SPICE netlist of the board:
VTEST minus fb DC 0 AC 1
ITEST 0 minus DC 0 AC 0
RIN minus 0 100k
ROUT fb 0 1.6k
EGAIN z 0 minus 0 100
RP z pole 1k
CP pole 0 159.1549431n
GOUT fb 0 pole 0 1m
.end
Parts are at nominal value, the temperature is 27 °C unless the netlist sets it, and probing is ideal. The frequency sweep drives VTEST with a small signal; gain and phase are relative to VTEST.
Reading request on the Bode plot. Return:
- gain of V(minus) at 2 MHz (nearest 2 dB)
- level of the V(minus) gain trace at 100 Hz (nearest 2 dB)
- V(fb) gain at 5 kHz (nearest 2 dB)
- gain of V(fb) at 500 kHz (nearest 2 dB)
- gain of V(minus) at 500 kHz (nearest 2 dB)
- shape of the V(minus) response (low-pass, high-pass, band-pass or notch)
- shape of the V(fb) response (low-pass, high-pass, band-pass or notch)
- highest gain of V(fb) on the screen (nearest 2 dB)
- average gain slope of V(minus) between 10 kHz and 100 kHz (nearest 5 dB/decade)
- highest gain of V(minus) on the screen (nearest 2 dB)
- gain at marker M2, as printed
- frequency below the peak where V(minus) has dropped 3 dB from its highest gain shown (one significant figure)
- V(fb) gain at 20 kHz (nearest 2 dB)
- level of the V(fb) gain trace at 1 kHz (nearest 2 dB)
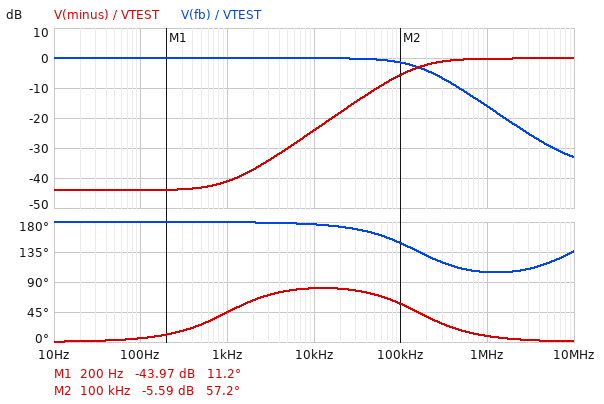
0 dB
-44 dB
0 dB
-10 dB
0 dB
high-pass
low-pass
0 dB
20 dB/decade
0 dB
-5.59 dB
200 kHz
0 dB
0 dB
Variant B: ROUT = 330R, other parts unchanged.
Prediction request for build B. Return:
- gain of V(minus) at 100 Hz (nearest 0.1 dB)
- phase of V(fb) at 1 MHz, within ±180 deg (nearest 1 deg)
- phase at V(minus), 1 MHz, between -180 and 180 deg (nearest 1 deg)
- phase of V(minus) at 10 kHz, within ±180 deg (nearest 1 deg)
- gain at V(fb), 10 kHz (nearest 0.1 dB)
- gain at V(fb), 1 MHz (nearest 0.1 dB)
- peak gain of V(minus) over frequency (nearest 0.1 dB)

-30.6 dB
98 deg
2 deg
68 deg
-0.6 dB
-29.6 dB
0 dB
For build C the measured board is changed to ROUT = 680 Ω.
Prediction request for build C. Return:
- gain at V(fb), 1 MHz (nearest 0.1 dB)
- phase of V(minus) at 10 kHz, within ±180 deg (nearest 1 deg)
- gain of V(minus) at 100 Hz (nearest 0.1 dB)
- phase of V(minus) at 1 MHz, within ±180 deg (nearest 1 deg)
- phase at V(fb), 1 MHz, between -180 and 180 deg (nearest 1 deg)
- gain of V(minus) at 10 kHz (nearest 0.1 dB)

-23.4 dB
76 deg
-36.7 dB
4 deg
100 deg
-16.8 dB
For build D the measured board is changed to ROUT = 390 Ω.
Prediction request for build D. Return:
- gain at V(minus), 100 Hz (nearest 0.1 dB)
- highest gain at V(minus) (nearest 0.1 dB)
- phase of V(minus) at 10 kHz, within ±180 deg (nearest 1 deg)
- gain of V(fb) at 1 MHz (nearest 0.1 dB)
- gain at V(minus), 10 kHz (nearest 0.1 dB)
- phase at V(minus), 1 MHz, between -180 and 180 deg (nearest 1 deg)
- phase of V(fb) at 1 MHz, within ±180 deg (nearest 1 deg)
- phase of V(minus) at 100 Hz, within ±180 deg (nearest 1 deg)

-32.0 dB
0 dB
70 deg
-28.2 dB
-12.3 dB
2 deg
98 deg
6 deg
